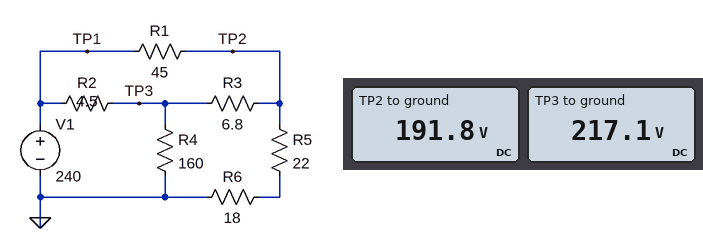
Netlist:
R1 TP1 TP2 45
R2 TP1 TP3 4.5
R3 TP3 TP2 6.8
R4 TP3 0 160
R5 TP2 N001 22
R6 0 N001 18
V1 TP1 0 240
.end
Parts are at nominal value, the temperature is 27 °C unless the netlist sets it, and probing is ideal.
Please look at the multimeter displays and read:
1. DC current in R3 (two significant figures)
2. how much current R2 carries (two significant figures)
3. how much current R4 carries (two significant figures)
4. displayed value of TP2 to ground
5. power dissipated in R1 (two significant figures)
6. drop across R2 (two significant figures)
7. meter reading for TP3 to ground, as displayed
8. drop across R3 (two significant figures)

3.7 A
5.1 A
1.4 A
191.8 V
52 W
23 V
217.1 V
25 V
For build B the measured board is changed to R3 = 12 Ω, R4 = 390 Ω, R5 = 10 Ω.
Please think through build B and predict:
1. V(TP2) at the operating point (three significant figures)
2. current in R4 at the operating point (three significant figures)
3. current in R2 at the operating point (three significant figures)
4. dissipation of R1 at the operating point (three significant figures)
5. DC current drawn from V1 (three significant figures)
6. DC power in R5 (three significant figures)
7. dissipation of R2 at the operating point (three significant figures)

166 V
559 mA
4.87 A
120 W
6.50 A
353 W
107 W
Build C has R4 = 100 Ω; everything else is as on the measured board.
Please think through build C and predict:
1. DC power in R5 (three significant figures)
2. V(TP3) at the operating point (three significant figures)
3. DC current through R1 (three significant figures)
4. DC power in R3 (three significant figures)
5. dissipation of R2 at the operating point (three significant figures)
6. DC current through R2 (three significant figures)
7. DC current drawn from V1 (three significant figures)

494 W
214 V
1.12 A
88.9 W
149 W
5.76 A
6.88 A
